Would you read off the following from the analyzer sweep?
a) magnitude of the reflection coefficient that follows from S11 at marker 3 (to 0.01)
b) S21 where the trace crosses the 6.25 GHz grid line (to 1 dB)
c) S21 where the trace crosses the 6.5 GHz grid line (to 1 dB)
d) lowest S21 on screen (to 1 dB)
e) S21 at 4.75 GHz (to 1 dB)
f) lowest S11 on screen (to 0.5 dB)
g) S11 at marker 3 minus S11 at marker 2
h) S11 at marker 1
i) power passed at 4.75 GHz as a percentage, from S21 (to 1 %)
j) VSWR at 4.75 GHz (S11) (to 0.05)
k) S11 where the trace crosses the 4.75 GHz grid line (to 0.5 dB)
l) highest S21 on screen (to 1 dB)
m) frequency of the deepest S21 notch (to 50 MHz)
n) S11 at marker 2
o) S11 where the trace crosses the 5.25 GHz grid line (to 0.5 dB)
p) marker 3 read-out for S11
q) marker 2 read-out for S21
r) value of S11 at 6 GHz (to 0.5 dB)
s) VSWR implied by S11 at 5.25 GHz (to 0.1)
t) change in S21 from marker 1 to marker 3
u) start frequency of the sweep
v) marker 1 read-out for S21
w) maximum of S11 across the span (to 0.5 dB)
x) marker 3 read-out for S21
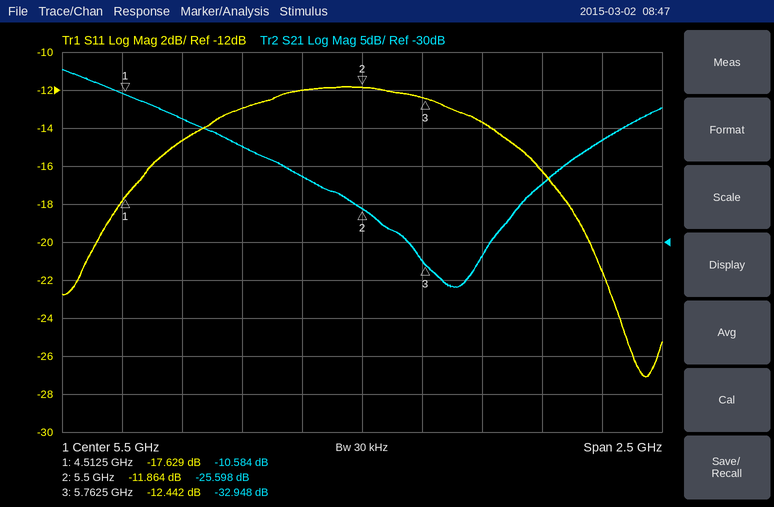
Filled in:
0.24
-22 dB
-17 dB
-36 dB
-14 dB
-27.0 dB
-0.578 dB
-17.629 dB
4 %
1.45
-14.5 dB
-7 dB
5.90 GHz
-11.864 dB
-12.0 dB
-12.442 dB
-25.598 dB
-13.5 dB
1.7
-22.364 dB
4.25 GHz
-10.584 dB
-12.0 dB
-32.948 dB
